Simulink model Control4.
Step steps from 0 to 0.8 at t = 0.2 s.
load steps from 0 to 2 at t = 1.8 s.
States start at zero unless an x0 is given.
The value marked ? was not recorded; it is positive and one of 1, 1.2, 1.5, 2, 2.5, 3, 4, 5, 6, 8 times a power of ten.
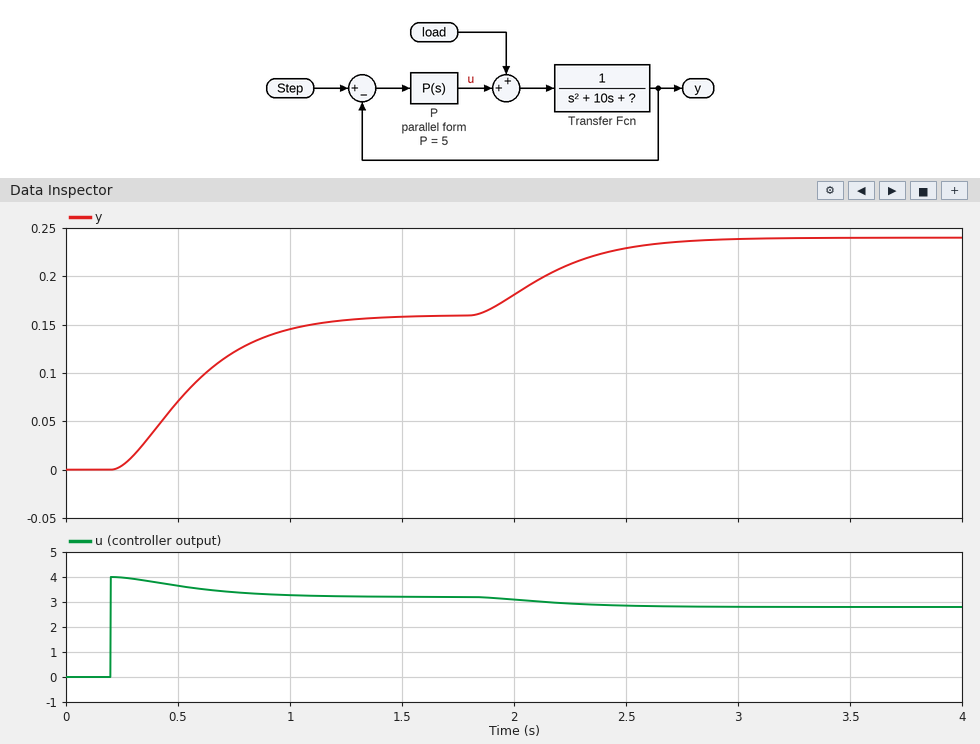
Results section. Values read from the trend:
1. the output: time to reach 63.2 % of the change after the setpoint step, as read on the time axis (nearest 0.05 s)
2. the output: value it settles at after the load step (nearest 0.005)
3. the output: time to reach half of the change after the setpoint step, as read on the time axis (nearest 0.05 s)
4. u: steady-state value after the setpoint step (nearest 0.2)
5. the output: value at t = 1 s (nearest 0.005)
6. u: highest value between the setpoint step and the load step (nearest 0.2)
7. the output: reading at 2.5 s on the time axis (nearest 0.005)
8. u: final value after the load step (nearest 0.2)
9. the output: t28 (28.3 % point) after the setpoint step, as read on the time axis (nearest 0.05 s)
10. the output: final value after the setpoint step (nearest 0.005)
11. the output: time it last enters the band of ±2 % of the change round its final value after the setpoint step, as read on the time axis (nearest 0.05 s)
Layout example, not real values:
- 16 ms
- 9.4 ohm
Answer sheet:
- 0.65 s
- 0.240
- 0.55 s
- 3.2
- 0.145
- 4.0
- 0.230
- 2.8
- 0.40 s
- 0.160
- 1.35 s
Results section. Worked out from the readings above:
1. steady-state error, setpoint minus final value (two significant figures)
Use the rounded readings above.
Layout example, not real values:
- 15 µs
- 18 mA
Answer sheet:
- 0.64
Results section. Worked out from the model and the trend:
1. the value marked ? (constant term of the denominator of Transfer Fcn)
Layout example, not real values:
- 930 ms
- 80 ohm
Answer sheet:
- 20
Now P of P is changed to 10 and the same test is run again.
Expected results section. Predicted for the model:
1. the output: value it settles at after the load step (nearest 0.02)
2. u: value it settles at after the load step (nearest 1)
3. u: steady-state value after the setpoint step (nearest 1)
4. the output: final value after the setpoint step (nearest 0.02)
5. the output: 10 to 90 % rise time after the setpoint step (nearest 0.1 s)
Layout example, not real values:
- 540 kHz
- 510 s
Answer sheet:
- 0.34
- 5
- 5
- 0.26
- 0.5 s
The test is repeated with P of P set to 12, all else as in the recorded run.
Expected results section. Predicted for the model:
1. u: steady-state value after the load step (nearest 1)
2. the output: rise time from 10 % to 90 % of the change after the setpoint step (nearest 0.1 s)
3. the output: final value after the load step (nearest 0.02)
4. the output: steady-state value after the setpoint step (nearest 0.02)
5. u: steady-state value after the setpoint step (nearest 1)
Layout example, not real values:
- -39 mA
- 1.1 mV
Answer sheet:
- 5
- 0.5 s
- 0.36
- 0.30
- 6
